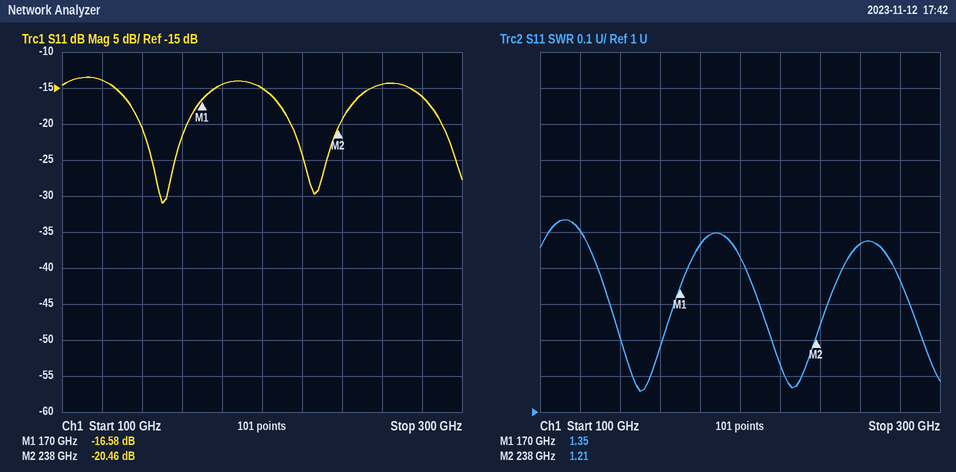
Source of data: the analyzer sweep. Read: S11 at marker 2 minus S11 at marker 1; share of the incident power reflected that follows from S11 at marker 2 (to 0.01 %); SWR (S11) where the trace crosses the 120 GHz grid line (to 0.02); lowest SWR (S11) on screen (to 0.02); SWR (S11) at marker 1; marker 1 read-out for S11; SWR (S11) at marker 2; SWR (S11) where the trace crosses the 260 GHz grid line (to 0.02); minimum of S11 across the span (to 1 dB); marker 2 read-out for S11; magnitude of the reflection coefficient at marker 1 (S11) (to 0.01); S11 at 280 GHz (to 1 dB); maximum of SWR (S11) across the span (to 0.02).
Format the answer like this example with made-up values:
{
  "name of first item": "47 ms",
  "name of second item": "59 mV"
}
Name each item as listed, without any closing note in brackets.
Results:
{
  "S11 at marker 2 minus S11 at marker 1": "-3.88 dB",
  "share of the incident power reflected that follows from S11 at marker 2": "0.90 %",
  "SWR (S11) where the trace crosses the 120 GHz grid line": "1.50",
  "lowest SWR (S11) on screen": "1.06",
  "SWR (S11) at marker 1": "1.35",
  "marker 1 read-out for S11": "-16.58 dB",
  "SWR (S11) at marker 2": "1.21",
  "SWR (S11) where the trace crosses the 260 GHz grid line": "1.46",
  "minimum of S11 across the span": "-31 dB",
  "marker 2 read-out for S11": "-20.46 dB",
  "magnitude of the reflection coefficient at marker 1 (S11)": "0.15",
  "S11 at 280 GHz": "-16 dB",
  "maximum of SWR (S11) across the span": "1.54"
}
